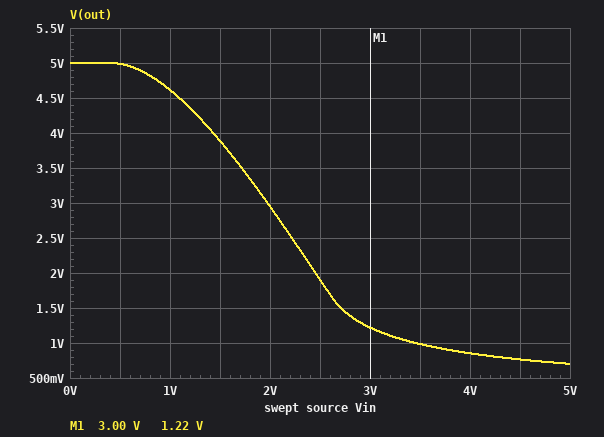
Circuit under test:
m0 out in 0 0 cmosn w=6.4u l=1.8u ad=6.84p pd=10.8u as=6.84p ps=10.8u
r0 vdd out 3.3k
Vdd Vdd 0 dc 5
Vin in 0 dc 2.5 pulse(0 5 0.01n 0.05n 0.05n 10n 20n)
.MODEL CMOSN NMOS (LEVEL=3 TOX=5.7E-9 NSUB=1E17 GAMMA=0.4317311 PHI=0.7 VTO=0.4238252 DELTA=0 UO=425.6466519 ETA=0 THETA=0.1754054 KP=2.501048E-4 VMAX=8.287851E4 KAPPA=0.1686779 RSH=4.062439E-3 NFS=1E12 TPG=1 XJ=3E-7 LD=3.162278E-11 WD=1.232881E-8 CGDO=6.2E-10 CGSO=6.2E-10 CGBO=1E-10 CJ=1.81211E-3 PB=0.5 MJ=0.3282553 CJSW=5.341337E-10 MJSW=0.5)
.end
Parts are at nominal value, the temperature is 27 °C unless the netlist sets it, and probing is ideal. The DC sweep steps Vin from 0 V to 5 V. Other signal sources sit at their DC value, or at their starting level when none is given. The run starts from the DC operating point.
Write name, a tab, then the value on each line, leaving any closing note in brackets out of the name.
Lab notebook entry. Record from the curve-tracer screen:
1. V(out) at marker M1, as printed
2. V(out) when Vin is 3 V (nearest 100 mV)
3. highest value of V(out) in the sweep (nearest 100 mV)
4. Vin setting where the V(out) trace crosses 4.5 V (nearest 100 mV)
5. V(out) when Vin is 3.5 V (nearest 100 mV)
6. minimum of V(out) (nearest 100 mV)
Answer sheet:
V(out) at marker M1, as printed	1.22 V
V(out) when Vin is 3 V	1.2 V
highest value of V(out) in the sweep	5.0 V
Vin setting where the V(out) trace crosses 4.5 V	1.1 V
V(out) when Vin is 3.5 V	1.0 V
minimum of V(out)	700 mV
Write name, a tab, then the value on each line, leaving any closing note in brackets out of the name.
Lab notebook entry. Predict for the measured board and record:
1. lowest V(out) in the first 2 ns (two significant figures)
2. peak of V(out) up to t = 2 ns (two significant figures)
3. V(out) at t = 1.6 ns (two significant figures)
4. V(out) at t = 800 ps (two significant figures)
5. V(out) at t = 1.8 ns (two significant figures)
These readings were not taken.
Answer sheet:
lowest V(out) in the first 2 ns	700 mV
peak of V(out) up to t = 2 ns	5.3 V
V(out) at t = 1.6 ns	700 mV
V(out) at t = 800 ps	700 mV
V(out) at t = 1.8 ns	700 mV
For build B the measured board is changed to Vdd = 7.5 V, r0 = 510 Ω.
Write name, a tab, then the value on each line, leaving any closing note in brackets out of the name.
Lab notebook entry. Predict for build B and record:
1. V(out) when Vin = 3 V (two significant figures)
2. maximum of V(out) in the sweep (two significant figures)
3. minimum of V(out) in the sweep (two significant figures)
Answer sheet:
V(out) when Vin = 3 V	6.8 V
maximum of V(out) in the sweep	7.5 V
minimum of V(out) in the sweep	6.0 V
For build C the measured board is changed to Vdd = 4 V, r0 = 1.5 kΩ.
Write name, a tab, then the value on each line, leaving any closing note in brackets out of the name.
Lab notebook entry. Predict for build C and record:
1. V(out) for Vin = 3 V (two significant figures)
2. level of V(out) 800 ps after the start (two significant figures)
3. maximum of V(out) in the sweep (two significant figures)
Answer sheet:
V(out) for Vin = 3 V	2.1 V
level of V(out) 800 ps after the start	1.2 V
maximum of V(out) in the sweep	4.0 V
